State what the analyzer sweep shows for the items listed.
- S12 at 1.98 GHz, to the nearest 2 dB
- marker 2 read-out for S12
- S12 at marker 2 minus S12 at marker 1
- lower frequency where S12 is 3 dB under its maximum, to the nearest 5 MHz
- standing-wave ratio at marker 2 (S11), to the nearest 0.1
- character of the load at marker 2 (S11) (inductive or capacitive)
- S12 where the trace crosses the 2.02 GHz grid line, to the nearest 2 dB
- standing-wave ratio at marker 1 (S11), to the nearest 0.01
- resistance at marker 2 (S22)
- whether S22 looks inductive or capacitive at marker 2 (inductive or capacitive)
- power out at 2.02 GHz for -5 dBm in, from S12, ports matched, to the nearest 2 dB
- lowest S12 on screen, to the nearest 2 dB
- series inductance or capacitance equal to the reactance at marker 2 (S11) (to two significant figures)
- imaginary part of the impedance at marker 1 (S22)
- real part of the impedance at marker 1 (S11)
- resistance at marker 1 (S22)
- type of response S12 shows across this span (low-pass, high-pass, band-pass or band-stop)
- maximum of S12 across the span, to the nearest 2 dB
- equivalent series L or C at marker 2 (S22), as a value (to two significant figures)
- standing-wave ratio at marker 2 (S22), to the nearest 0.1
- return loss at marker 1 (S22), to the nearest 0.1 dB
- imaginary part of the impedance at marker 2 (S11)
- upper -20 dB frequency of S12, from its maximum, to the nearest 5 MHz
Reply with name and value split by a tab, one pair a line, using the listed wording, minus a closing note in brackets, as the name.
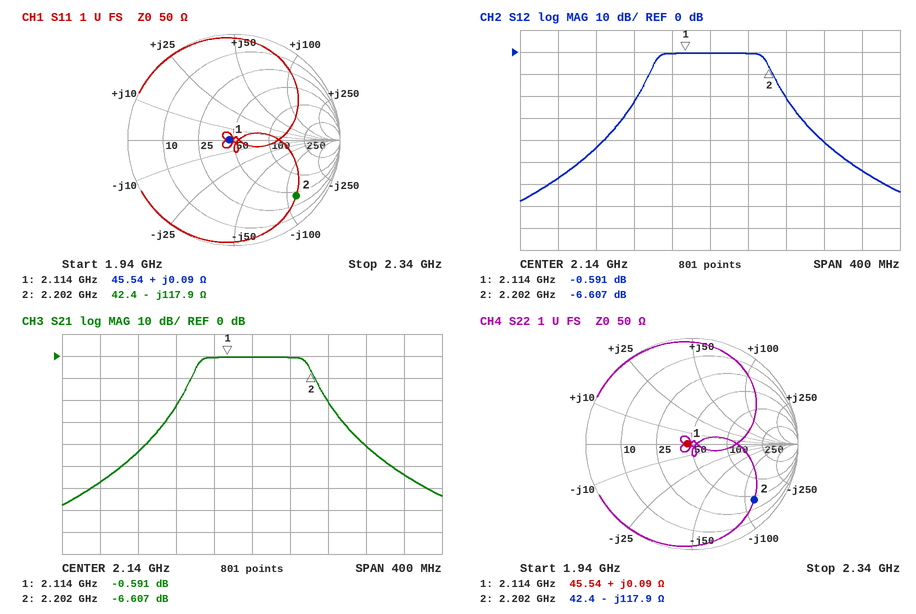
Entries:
S12 at 1.98 GHz, to the nearest 2 dB	-58 dB
marker 2 read-out for S12	-6.607 dB
S12 at marker 2 minus S12 at marker 1	-6.016 dB
lower frequency where S12 is 3 dB under its maximum, to the nearest 5 MHz	2.085 GHz
standing-wave ratio at marker 2 (S11), to the nearest 0.1	8.5
character of the load at marker 2 (S11)	capacitive
S12 where the trace crosses the 2.02 GHz grid line, to the nearest 2 dB	-44 dB
standing-wave ratio at marker 1 (S11), to the nearest 0.01	1.10
resistance at marker 2	42.4 Ω
whether S22 looks inductive or capacitive at marker 2	capacitive
power out at 2.02 GHz for -5 dBm in, from S12, ports matched, to the nearest 2 dB	-48 dBm
lowest S12 on screen, to the nearest 2 dB	-68 dB
series inductance or capacitance equal to the reactance at marker 2 (S11)	610 fF
imaginary part of the impedance at marker 1	+0.09 Ω
real part of the impedance at marker 1	45.54 Ω
resistance at marker 1	45.54 Ω
type of response S12 shows across this span	band-pass
maximum of S12 across the span, to the nearest 2 dB	0 dB
equivalent series L or C at marker 2 (S22), as a value	610 fF
standing-wave ratio at marker 2 (S22), to the nearest 0.1	8.5
return loss at marker 1 (S22), to the nearest 0.1 dB	26.6 dB
imaginary part of the impedance at marker 2	-117.9 Ω
upper -20 dB frequency of S12, from its maximum, to the nearest 5 MHz	2.220 GHz
